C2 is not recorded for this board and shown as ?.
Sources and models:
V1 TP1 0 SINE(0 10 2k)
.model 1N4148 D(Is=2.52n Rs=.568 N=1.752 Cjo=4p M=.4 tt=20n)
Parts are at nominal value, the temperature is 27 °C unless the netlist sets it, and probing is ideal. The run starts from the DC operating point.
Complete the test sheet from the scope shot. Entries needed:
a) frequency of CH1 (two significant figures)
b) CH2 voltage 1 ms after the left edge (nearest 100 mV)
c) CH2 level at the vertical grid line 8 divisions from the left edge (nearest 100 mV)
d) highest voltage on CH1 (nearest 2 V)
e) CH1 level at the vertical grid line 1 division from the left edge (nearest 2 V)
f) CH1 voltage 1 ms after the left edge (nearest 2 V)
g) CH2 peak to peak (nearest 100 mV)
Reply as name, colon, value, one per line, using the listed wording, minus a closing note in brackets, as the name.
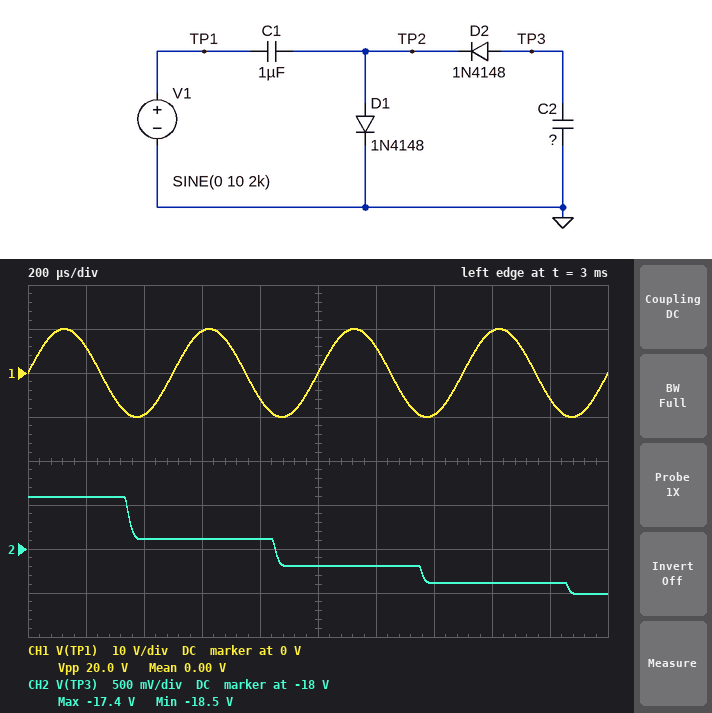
frequency of CH1: 2.0 kHz
CH2 voltage 1 ms after the left edge: -18.2 V
CH2 level at the vertical grid line 8 divisions from the left edge: -18.4 V
highest voltage on CH1: 10 V
CH1 level at the vertical grid line 1 division from the left edge: 6 V
CH1 voltage 1 ms after the left edge: 0 V
CH2 peak to peak: 1.1 V
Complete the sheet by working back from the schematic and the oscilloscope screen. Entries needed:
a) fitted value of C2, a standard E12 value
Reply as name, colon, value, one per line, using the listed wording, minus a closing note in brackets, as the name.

fitted value of C2, a standard E12 value: 1.8 µF
